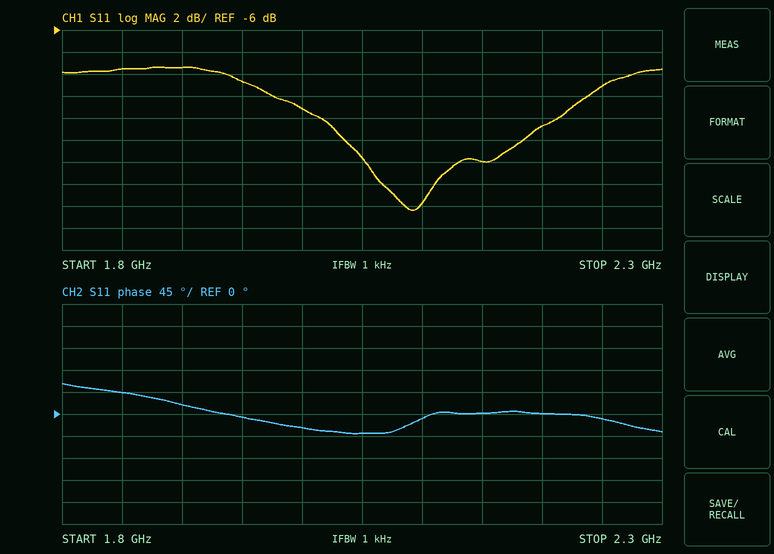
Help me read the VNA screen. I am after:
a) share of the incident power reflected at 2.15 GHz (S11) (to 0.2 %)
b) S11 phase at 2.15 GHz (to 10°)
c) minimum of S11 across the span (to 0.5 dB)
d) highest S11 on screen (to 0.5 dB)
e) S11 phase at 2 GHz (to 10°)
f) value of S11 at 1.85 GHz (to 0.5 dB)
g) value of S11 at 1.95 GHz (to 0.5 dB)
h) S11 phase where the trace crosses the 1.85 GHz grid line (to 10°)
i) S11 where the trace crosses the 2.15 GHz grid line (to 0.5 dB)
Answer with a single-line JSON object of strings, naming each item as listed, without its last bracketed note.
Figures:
{"share of the incident power reflected at 2.15 GHz (S11)": "1.6 %", "S11 phase at 2.15 GHz": "0°", "minimum of S11 across the span": "-22.5 dB", "highest S11 on screen": "-9.5 dB", "S11 phase at 2 GHz": "-30°", "value of S11 at 1.85 GHz": "-9.5 dB", "value of S11 at 1.95 GHz": "-10.5 dB", "S11 phase where the trace crosses the 1.85 GHz grid line": "40°", "S11 where the trace crosses the 2.15 GHz grid line": "-18.0 dB"}
